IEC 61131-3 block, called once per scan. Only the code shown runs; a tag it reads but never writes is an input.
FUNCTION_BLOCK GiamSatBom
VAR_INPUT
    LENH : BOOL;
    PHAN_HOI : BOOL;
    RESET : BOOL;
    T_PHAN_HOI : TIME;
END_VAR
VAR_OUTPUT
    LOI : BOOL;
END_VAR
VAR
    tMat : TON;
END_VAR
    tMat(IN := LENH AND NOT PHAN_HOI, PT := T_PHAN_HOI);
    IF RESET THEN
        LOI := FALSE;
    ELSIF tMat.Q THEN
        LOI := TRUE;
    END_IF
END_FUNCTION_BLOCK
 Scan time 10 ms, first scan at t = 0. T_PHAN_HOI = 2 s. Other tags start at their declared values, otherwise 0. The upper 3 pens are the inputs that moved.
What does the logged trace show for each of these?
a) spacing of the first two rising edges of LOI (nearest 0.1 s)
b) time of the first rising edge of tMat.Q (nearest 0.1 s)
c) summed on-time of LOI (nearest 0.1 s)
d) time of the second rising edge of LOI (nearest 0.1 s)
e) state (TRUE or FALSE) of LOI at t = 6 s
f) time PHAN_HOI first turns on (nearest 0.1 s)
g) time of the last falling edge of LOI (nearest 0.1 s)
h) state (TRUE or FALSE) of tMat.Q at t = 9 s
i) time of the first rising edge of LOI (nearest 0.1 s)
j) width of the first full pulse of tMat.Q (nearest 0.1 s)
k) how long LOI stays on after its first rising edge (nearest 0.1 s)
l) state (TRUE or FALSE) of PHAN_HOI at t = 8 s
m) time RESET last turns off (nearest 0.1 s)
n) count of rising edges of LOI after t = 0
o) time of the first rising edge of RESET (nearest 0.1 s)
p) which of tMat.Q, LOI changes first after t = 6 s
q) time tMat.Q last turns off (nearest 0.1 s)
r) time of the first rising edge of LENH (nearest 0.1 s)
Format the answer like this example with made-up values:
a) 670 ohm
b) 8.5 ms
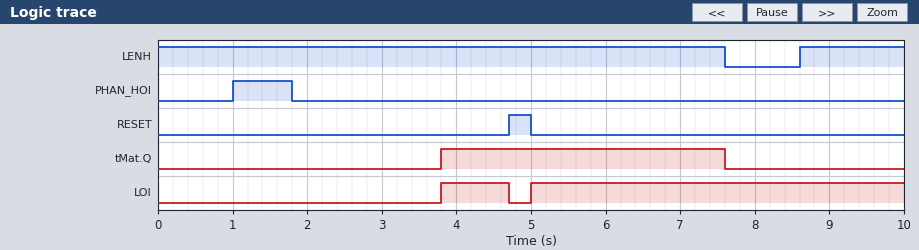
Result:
a) 1.2 s
b) 3.8 s
c) 5.9 s
d) 5.0 s
e) TRUE
f) 1.0 s
g) 4.7 s
h) FALSE
i) 3.8 s
j) 3.8 s
k) 0.9 s
l) FALSE
m) 5.0 s
n) 2
o) 4.7 s
p) tMat.Q
q) 7.6 s
r) 8.6 s
